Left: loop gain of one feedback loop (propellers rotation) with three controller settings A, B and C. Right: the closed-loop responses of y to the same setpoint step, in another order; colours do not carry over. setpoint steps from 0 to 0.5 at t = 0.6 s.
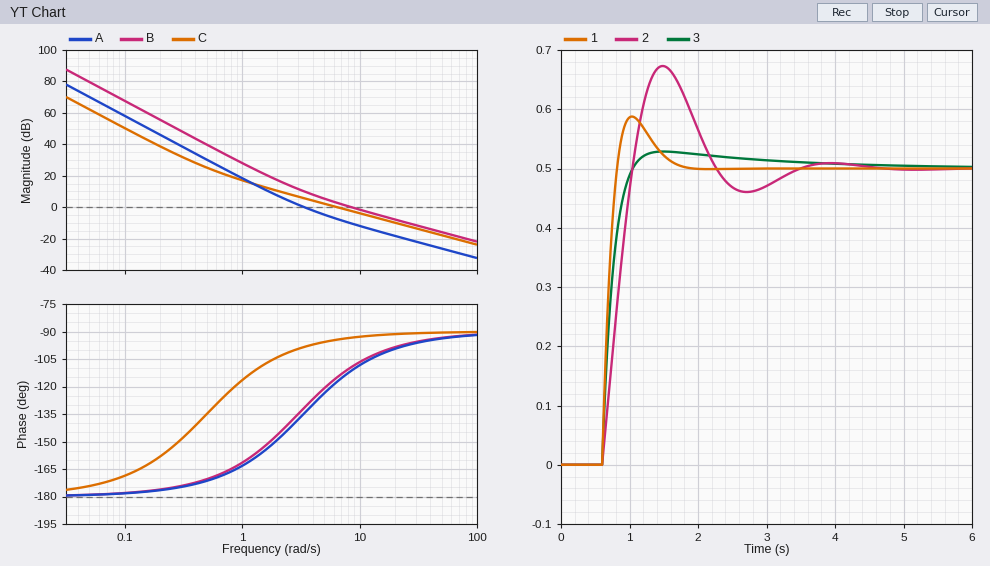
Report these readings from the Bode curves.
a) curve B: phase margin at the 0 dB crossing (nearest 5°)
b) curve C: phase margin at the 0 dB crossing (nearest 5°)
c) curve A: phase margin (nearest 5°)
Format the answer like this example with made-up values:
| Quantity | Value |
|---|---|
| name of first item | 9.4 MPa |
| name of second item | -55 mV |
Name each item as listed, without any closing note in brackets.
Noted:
| Quantity | Value |
|---|---|
| curve B: phase margin at the 0 dB crossing | 70° |
| curve C: phase margin at the 0 dB crossing | 85° |
| curve A: phase margin | 45° |
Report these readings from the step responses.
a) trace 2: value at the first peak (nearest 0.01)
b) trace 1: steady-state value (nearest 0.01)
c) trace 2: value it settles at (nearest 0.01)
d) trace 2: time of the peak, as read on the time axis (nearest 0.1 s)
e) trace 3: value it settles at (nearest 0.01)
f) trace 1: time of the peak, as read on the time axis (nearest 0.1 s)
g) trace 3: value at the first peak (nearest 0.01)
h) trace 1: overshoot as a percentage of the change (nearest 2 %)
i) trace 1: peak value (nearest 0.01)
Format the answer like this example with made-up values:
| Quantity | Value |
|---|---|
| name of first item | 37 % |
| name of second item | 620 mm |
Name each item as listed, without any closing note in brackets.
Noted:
| Quantity | Value |
|---|---|
| trace 2: value at the first peak | 0.67 |
| trace 1: steady-state value | 0.50 |
| trace 2: value it settles at | 0.50 |
| trace 2: time of the peak, as read on the time axis | 1.5 s |
| trace 3: value it settles at | 0.50 |
| trace 1: time of the peak, as read on the time axis | 1.0 s |
| trace 3: value at the first peak | 0.53 |
| trace 1: overshoot as a percentage of the change | 18 % |
| trace 1: peak value | 0.59 |
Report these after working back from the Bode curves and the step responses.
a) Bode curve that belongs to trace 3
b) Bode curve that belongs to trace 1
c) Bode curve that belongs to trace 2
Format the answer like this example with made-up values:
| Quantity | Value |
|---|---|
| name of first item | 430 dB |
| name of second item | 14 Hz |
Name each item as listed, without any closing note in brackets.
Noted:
| Quantity | Value |
|---|---|
| Bode curve that belongs to trace 3 | C |
| Bode curve that belongs to trace 1 | B |
| Bode curve that belongs to trace 2 | A |
